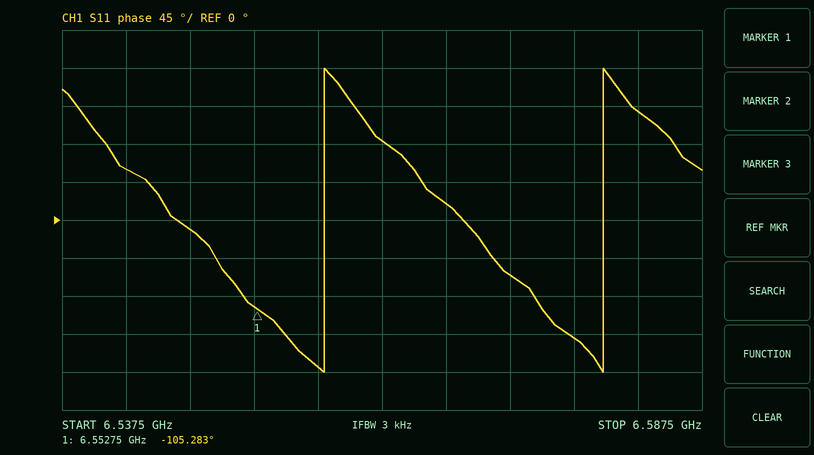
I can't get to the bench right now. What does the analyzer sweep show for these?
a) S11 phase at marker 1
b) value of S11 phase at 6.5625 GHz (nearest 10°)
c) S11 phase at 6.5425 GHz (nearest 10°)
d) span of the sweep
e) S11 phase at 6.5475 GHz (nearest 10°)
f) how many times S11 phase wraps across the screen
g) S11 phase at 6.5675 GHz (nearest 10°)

-105.283°
90°
60°
50 MHz
-10°
2
20°
